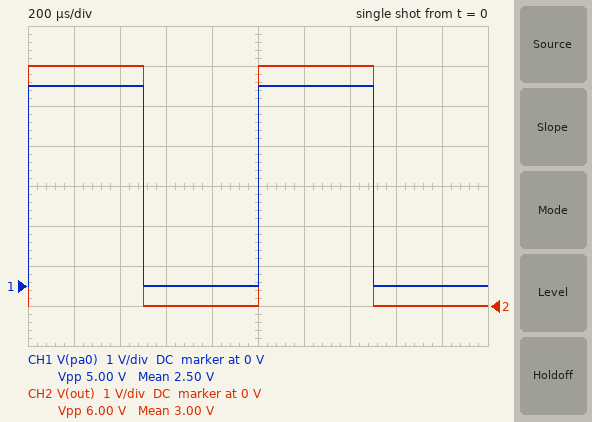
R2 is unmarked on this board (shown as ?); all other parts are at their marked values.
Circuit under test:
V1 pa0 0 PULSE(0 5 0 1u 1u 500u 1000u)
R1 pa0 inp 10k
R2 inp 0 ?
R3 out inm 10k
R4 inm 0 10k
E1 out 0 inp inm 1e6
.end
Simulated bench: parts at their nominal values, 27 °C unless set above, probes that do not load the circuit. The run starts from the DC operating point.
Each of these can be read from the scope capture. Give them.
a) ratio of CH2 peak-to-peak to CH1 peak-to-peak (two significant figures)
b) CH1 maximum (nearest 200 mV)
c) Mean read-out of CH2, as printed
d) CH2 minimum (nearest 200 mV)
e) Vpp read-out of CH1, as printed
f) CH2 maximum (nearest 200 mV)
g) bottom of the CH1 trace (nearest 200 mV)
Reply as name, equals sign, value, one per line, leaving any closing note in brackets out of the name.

ratio of CH2 peak-to-peak to CH1 peak-to-peak = 1.2
CH1 maximum = 5.0 V
Mean read-out of CH2, as printed = 3.00 V
CH2 minimum = 0 V
Vpp read-out of CH1, as printed = 5.00 V
CH2 maximum = 6.0 V
bottom of the CH1 trace = 0 V
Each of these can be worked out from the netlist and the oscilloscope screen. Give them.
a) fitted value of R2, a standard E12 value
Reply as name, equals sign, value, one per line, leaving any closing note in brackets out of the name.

fitted value of R2, a standard E12 value = 15 kΩ
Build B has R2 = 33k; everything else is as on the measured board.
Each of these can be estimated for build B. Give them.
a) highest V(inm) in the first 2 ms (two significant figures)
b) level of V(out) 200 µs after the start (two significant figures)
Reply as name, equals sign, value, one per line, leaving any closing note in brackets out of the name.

highest V(inm) in the first 2 ms = 3.8 V
level of V(out) 200 µs after the start = 7.7 V
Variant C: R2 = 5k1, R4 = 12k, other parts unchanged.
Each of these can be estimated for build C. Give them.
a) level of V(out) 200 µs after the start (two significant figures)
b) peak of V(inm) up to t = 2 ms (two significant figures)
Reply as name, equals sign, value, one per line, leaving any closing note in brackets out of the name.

level of V(out) 200 µs after the start = 3.1 V
peak of V(inm) up to t = 2 ms = 1.7 V
